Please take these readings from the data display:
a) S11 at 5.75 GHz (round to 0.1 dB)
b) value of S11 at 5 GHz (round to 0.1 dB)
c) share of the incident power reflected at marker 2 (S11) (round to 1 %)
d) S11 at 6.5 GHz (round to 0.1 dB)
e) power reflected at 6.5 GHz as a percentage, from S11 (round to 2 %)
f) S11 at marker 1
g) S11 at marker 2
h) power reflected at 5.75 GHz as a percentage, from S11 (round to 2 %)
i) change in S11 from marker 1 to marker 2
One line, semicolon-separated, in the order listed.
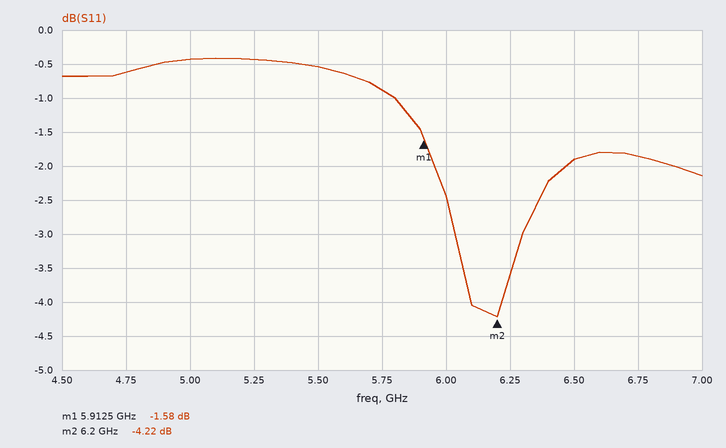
-0.9 dB; -0.4 dB; 38 %; -1.9 dB; 64 %; -1.58 dB; -4.22 dB; 82 %; -2.64 dB
